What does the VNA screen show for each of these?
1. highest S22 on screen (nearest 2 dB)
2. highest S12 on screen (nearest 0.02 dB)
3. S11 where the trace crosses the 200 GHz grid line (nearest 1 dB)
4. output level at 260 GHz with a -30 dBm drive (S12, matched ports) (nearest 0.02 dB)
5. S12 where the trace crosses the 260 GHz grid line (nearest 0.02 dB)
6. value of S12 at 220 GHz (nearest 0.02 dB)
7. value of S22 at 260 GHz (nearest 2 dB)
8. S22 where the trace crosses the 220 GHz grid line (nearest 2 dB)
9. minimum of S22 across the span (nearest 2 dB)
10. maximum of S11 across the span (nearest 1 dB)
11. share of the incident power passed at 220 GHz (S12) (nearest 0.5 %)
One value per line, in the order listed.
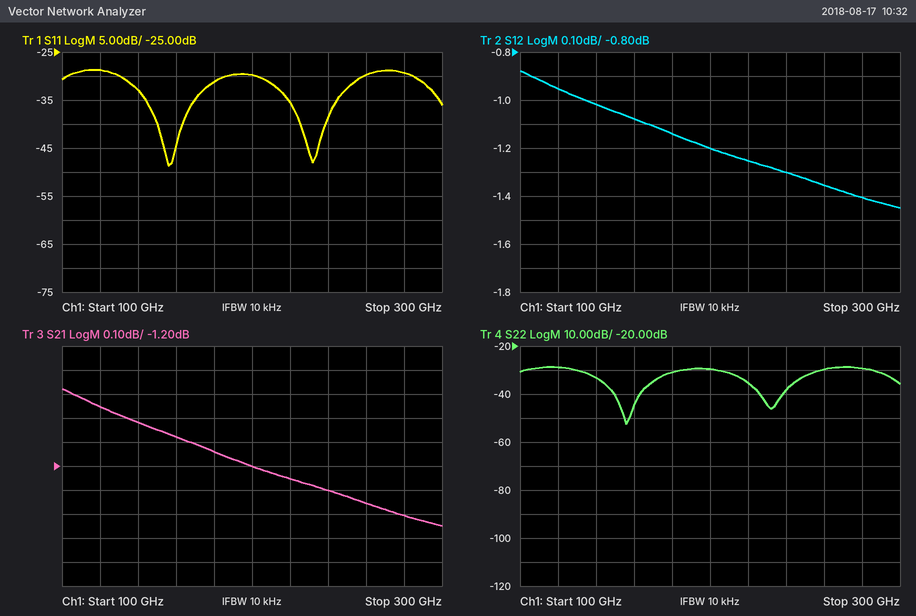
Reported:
-28 dB
-0.88 dB
-30 dB
-31.36 dBm
-1.36 dB
-1.26 dB
-30 dB
-36 dB
-52 dB
-29 dB
75.0 %
